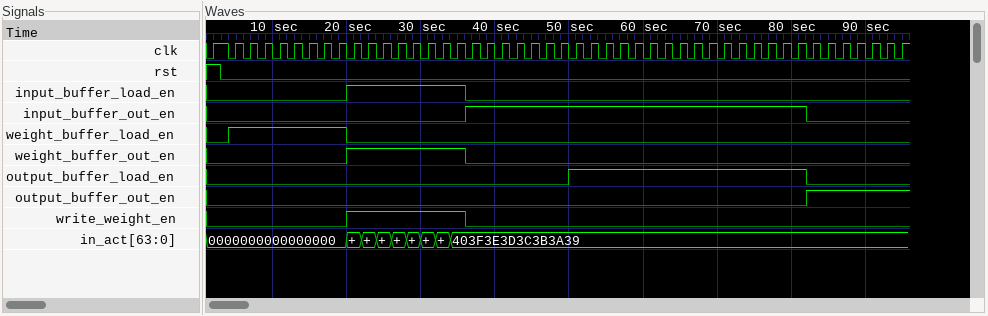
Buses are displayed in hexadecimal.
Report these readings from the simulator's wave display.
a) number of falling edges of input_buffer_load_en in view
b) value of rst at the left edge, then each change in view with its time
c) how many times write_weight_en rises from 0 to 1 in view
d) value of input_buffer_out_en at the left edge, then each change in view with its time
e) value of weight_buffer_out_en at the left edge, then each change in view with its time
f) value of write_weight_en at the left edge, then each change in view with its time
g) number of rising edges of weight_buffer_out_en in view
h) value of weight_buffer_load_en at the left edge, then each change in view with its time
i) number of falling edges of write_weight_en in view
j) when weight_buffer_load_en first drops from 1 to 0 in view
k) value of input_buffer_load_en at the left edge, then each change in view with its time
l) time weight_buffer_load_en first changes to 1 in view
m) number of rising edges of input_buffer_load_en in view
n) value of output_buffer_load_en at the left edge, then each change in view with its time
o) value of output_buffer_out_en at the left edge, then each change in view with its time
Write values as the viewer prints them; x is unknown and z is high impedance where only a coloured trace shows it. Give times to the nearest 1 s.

1
1, 0 at 3 s
1
0, 1 at 36 s, 0 at 82 s
0, 1 at 20 s, 0 at 36 s
0, 1 at 20 s, 0 at 36 s
1
0, 1 at 4 s, 0 at 20 s
1
20 s
0, 1 at 20 s, 0 at 36 s
4 s
1
0, 1 at 50 s, 0 at 82 s
0, 1 at 82 s
